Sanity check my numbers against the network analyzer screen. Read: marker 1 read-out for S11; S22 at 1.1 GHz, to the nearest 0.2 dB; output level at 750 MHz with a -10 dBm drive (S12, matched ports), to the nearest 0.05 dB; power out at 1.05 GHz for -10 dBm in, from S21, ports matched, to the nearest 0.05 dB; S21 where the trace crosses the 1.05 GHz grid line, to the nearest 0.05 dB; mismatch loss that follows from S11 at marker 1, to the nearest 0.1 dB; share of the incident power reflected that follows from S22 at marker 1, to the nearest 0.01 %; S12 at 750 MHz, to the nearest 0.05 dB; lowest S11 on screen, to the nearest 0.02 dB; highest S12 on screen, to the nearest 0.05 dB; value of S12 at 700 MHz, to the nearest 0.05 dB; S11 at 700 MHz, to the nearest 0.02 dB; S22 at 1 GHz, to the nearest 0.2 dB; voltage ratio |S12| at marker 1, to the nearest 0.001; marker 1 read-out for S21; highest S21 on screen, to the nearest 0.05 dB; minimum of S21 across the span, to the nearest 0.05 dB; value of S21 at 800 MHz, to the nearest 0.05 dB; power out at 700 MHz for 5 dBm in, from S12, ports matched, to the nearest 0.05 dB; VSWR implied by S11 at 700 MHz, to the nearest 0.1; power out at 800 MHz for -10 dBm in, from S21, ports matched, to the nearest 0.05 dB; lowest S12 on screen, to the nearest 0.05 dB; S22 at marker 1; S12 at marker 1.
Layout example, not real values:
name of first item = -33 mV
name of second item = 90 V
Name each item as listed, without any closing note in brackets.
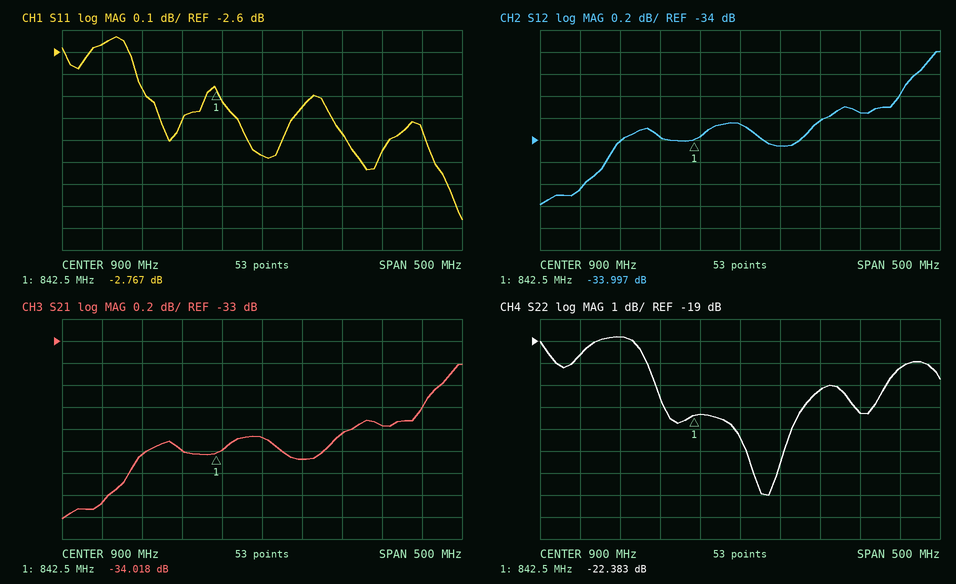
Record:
marker 1 read-out for S11 = -2.767 dB
S22 at 1.1 GHz, to the nearest 0.2 dB = -20.2 dB
output level at 750 MHz with a -10 dBm drive (S12, matched ports), to the nearest 0.05 dB = -44.00 dBm
power out at 1.05 GHz for -10 dBm in, from S21, ports matched, to the nearest 0.05 dB = -43.75 dBm
S21 where the trace crosses the 1.05 GHz grid line, to the nearest 0.05 dB = -33.75 dB
mismatch loss that follows from S11 at marker 1, to the nearest 0.1 dB = 3.3 dB
share of the incident power reflected that follows from S22 at marker 1, to the nearest 0.01 % = 0.58 %
S12 at 750 MHz, to the nearest 0.05 dB = -34.00 dB
lowest S11 on screen, to the nearest 0.02 dB = -3.36 dB
highest S12 on screen, to the nearest 0.05 dB = -33.20 dB
value of S12 at 700 MHz, to the nearest 0.05 dB = -34.45 dB
S11 at 700 MHz, to the nearest 0.02 dB = -2.56 dB
S22 at 1 GHz, to the nearest 0.2 dB = -21.2 dB
voltage ratio |S12| at marker 1, to the nearest 0.001 = 0.020
marker 1 read-out for S21 = -34.018 dB
highest S21 on screen, to the nearest 0.05 dB = -33.20 dB
minimum of S21 across the span, to the nearest 0.05 dB = -34.60 dB
value of S21 at 800 MHz, to the nearest 0.05 dB = -34.00 dB
power out at 700 MHz for 5 dBm in, from S12, ports matched, to the nearest 0.05 dB = -29.45 dBm
VSWR implied by S11 at 700 MHz, to the nearest 0.1 = 6.8
power out at 800 MHz for -10 dBm in, from S21, ports matched, to the nearest 0.05 dB = -44.00 dBm
lowest S12 on screen, to the nearest 0.05 dB = -34.60 dB
S22 at marker 1 = -22.383 dB
S12 at marker 1 = -33.997 dB
